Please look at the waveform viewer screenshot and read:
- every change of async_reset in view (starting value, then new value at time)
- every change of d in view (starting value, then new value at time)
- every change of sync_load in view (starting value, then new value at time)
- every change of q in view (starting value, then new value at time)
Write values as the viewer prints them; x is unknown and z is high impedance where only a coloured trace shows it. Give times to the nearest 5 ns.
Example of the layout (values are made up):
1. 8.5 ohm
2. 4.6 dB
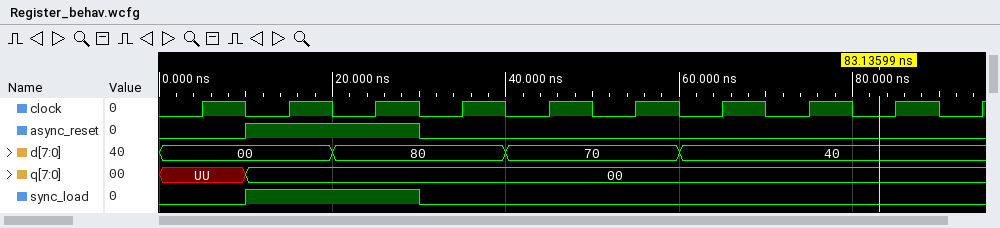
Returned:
1. 0, 1 at 10 ns, 0 at 30 ns
2. 00, 80 at 20 ns, 70 at 40 ns, 40 at 60 ns
3. 0, 1 at 10 ns, 0 at 30 ns
4. UU, 00 at 10 ns
